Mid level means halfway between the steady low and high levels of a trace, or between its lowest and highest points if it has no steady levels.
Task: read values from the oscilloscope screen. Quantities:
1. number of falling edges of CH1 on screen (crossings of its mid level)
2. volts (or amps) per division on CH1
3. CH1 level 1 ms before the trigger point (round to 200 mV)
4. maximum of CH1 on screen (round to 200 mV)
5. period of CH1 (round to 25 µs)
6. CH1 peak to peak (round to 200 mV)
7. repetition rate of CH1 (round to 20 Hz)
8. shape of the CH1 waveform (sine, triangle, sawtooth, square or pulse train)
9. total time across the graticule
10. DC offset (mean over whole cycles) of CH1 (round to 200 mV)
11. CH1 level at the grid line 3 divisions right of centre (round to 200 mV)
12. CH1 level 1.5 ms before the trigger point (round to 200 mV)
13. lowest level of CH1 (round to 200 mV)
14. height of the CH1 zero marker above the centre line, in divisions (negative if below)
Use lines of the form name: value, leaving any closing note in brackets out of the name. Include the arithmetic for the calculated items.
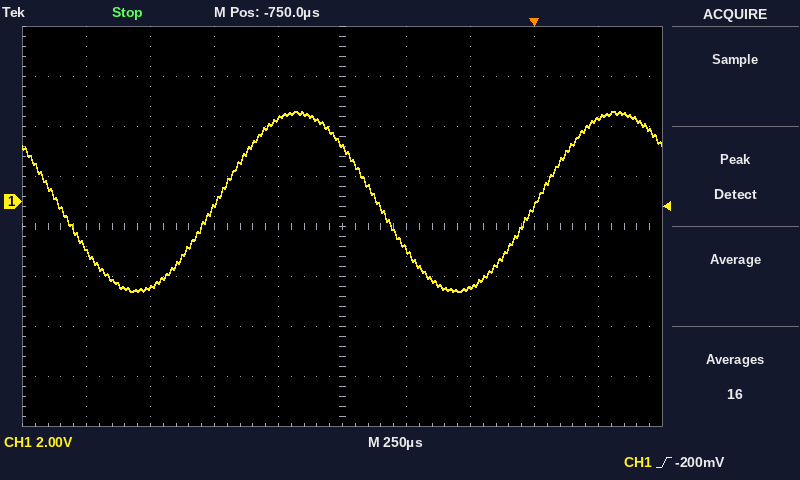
number of falling edges of CH1 on screen: 2
volts (or amps) per division on CH1: 2 V
CH1 level 1 ms before the trigger point: 3.4 V
maximum of CH1 on screen: 3.6 V
period of CH1: 1.250 ms
CH1 peak to peak: 3.6 V − (-3.6 V) = 7.2 V
repetition rate of CH1: 1 / 1.250 ms ≈ 800 Hz
shape of the CH1 waveform: sine
total time across the graticule: 2.5 ms
DC offset (mean over whole cycles) of CH1: (3.6 V + (-3.6 V)) / 2 ≈ 0.0 V
CH1 level at the grid line 3 divisions right of centre: -200 mV
CH1 level 1.5 ms before the trigger point: -3.4 V
lowest level of CH1: -3.6 V
height of the CH1 zero marker above the centre line, in divisions: +0.5 div
